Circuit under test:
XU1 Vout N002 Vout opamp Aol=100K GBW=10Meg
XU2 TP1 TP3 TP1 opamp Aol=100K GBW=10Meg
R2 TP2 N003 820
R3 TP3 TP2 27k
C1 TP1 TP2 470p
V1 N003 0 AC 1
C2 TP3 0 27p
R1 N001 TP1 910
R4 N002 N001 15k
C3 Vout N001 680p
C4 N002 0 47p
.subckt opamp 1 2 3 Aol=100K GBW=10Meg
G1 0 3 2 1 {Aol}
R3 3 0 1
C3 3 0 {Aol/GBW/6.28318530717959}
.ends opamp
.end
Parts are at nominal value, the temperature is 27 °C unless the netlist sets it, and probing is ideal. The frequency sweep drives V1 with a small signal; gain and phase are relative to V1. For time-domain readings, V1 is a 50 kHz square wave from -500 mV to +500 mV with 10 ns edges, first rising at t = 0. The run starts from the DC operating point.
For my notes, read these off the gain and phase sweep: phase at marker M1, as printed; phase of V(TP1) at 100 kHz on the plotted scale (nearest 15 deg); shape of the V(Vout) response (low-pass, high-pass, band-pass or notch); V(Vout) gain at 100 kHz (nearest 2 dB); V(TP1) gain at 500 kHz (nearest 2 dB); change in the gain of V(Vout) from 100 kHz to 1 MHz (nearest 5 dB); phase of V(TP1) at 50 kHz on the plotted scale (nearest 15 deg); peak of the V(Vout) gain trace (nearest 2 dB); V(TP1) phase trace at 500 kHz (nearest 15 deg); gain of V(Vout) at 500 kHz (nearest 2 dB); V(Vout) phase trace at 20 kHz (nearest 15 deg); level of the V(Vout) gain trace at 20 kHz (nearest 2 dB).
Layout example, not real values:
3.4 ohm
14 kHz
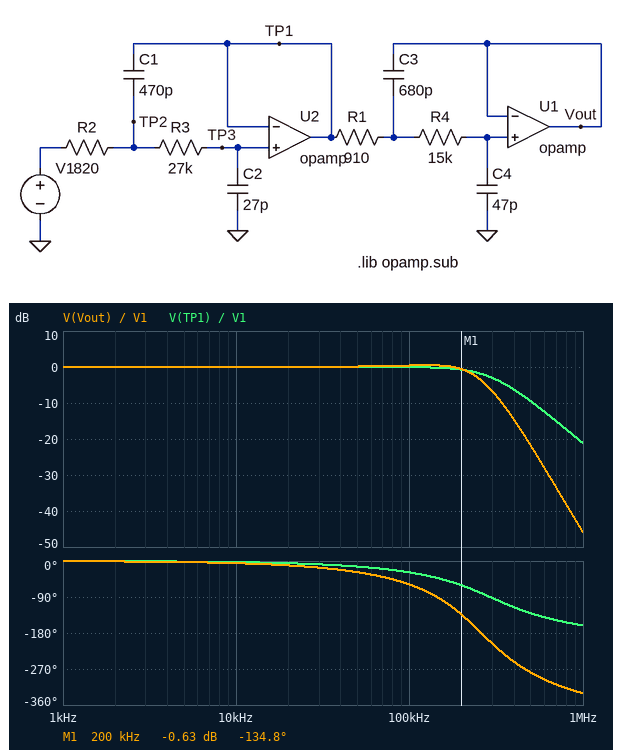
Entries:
-134.8 deg
-30 deg
low-pass
0 dB
-10 dB
-45 dB
-15 deg
0 dB
-135 deg
-22 dB
-15 deg
0 dB
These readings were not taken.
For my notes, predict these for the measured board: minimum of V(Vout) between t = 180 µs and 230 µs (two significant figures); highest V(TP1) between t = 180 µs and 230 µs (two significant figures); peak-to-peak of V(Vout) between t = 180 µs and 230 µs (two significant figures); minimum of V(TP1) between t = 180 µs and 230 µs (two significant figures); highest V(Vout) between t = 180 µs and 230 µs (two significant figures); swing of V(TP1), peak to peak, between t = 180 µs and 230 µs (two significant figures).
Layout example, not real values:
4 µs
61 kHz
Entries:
-630 mV
550 mV
1.3 V
-550 mV
630 mV
1.1 V
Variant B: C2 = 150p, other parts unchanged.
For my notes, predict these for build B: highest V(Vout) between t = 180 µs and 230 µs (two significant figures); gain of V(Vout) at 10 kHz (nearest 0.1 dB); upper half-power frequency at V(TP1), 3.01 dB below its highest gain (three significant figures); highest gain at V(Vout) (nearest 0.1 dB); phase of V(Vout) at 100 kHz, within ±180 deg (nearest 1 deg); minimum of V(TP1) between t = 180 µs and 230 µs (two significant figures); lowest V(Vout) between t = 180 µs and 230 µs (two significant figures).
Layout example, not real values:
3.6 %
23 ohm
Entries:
420 mV
-0.2 dB
41.9 kHz
0 dB
-113 deg
-430 mV
-420 mV
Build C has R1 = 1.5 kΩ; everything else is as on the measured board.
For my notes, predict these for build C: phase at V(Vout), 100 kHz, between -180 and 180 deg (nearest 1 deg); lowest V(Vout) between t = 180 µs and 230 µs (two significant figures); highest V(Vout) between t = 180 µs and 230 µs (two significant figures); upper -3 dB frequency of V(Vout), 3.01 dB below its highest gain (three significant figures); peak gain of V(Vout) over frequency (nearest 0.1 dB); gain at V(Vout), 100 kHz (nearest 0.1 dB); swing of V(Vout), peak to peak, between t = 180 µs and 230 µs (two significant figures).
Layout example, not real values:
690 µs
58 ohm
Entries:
-64 deg
-710 mV
710 mV
209 kHz
1.7 dB
1.3 dB
1.4 V
